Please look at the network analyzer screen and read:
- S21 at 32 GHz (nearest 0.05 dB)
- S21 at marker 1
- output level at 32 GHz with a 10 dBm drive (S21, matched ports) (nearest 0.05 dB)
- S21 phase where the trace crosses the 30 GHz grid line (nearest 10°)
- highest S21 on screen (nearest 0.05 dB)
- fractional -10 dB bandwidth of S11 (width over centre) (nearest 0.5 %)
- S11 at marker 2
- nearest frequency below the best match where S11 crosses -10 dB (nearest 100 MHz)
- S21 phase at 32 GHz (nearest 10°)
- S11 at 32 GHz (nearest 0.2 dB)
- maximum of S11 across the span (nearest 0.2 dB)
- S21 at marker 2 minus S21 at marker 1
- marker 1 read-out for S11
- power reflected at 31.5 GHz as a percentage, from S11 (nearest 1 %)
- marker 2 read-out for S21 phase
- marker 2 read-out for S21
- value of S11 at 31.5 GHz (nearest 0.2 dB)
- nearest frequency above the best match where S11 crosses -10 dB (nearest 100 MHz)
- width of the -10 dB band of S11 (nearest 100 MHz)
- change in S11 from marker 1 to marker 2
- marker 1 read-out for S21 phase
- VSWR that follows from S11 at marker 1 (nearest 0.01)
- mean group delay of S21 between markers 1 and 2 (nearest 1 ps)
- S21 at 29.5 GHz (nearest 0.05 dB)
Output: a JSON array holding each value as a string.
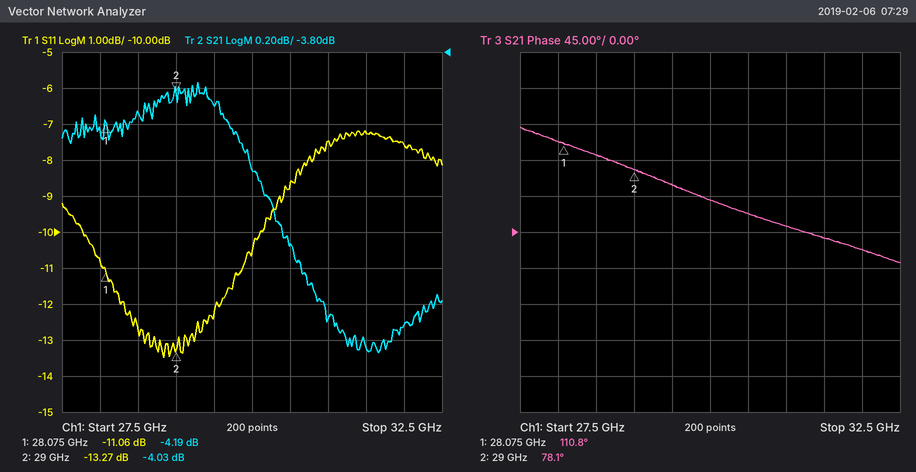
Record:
["-5.30 dB", "-4.19 dB", "4.70 dBm", "40°", "-3.95 dB", "8.0 %", "-13.27 dB", "27.8 GHz", "-20°", "-7.6 dB", "-7.2 dB", "0.16 dB", "-11.06 dB", "19 %", "78.1°", "-4.03 dB", "-7.2 dB", "30.1 GHz", "2.3 GHz", "-2.21 dB", "110.8°", "1.78", "98 ps", "-4.10 dB"]
